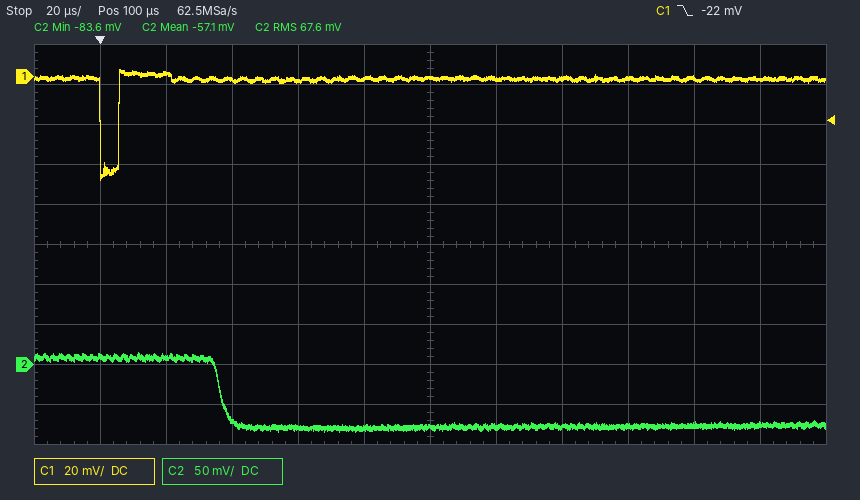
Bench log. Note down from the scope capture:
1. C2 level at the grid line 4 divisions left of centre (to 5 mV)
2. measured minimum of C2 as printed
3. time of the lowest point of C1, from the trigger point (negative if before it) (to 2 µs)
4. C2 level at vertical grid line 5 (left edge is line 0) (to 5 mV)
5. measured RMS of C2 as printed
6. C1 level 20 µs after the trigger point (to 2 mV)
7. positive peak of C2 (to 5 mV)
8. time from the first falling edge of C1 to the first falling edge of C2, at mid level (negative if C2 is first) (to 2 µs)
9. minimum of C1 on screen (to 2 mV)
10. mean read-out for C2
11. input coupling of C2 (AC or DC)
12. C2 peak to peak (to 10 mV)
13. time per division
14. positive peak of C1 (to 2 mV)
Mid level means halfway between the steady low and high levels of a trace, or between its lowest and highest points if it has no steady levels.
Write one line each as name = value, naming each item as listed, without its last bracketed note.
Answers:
C2 level at the grid line 4 divisions left of centre = 10 mV
measured minimum of C2 as printed = -83.6 mV
time of the lowest point of C1, from the trigger point (negative if before it) = 0 µs
C2 level at vertical grid line 5 (left edge is line 0) = -80 mV
measured RMS of C2 as printed = 67.6 mV
C1 level 20 µs after the trigger point = 2 mV
positive peak of C2 = 15 mV
time from the first falling edge of C1 to the first falling edge of C2, at mid level (negative if C2 is first) = +36 µs
minimum of C1 on screen = -52 mV
mean read-out for C2 = -57.1 mV
input coupling of C2 = DC
C2 peak to peak = 100 mV
time per division = 20 µs
positive peak of C1 = 4 mV
